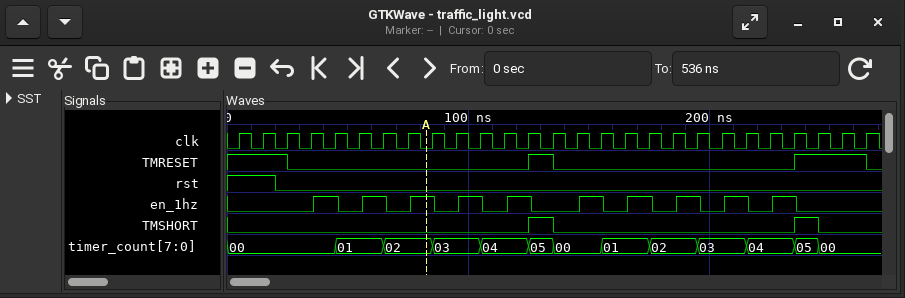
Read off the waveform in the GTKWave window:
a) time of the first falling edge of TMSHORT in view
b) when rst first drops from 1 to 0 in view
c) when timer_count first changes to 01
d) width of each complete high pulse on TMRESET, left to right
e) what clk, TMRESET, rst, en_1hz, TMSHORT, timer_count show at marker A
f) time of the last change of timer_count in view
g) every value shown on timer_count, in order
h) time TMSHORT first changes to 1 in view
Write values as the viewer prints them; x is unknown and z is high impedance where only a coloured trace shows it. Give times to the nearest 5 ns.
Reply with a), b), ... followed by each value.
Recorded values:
a) 135 ns
b) 20 ns
c) 45 ns
d) 10 ns, 30 ns
e) clk=0, TMRESET=0, rst=0, en_1hz=1, TMSHORT=0, timer_count=02
f) 245 ns
g) 00, 01, 02, 03, 04, 05, 00, 01, 02, 03, 04, 05, 00
h) 125 ns
